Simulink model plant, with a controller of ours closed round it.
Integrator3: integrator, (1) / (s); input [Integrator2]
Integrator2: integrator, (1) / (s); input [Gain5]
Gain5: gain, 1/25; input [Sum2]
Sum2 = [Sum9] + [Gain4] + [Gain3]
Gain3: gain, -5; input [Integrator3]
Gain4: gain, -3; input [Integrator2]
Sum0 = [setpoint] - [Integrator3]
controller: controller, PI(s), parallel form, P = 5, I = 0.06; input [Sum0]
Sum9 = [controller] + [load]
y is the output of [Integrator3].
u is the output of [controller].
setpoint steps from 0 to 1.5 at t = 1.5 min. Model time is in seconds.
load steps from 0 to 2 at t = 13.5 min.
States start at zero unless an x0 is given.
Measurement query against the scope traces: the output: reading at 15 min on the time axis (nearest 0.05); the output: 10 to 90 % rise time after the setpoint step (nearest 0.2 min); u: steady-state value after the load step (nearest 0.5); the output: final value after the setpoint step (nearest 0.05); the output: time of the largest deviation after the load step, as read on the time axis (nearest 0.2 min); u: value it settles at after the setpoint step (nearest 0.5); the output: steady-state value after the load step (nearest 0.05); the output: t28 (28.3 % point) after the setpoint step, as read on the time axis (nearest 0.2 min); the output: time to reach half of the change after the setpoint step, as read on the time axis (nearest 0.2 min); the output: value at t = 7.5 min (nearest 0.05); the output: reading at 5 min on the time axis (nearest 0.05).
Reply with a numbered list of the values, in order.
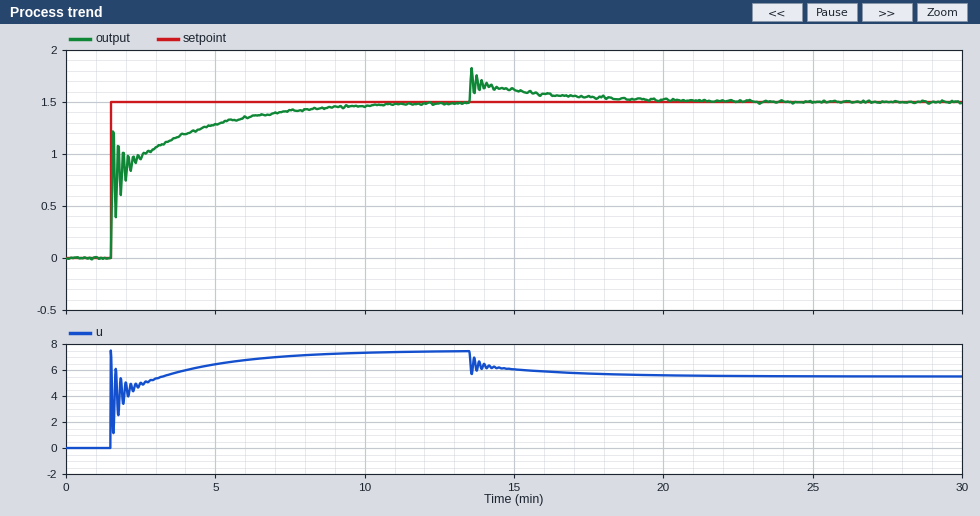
1. 1.60
2. 4.4 min
3. 5.5
4. 1.50
5. 13.6 min
6. 7.5
7. 1.50
8. 1.6 min
9. 1.6 min
10. 1.40
11. 1.30
